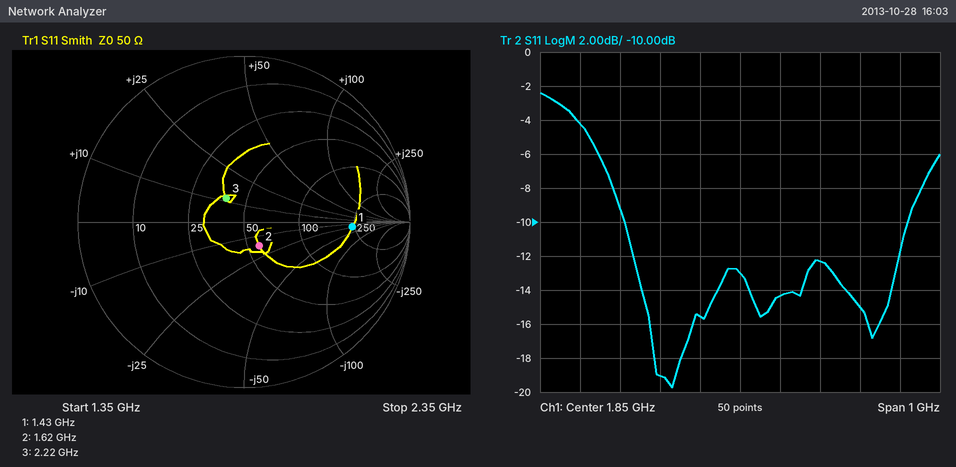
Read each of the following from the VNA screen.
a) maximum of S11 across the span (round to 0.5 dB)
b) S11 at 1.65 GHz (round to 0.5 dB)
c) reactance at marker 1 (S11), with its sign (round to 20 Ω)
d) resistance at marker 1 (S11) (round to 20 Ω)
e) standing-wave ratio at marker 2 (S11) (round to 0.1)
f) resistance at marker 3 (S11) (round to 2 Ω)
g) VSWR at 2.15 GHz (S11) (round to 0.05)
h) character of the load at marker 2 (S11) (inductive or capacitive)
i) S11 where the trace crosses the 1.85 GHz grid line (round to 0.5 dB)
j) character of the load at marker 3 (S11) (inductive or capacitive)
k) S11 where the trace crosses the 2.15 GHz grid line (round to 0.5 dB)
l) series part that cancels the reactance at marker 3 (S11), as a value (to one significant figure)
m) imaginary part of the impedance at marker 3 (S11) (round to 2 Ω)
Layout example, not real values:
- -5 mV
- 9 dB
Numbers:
- -2.5 dB
- -19.0 dB
- -20 Ω
- 240 Ω
- 1.4
- 38 Ω
- 1.45
- capacitive
- -13.0 dB
- inductive
- -15.0 dB
- 6 pF
- +12 Ω
